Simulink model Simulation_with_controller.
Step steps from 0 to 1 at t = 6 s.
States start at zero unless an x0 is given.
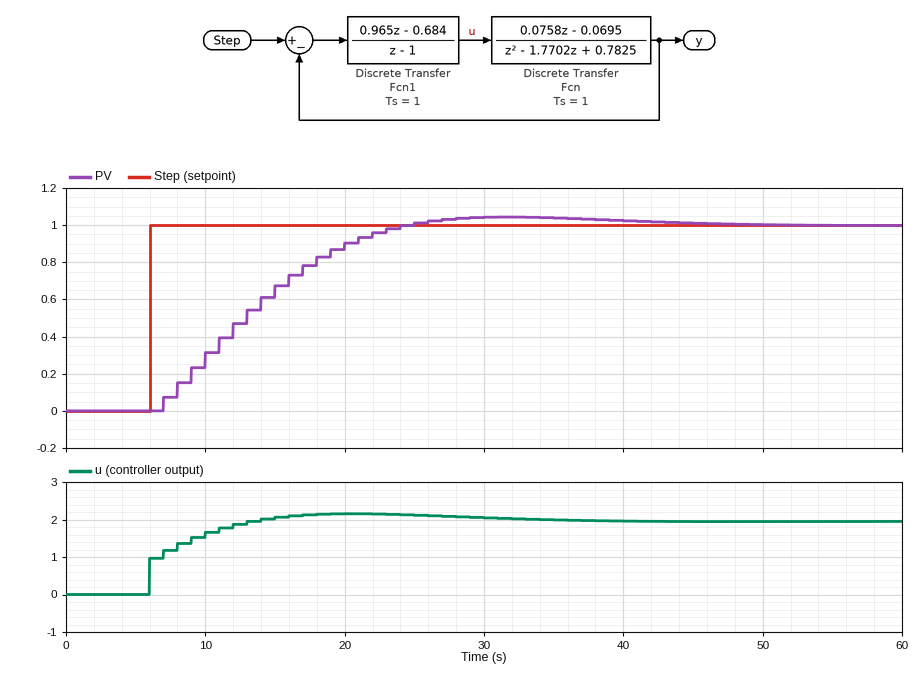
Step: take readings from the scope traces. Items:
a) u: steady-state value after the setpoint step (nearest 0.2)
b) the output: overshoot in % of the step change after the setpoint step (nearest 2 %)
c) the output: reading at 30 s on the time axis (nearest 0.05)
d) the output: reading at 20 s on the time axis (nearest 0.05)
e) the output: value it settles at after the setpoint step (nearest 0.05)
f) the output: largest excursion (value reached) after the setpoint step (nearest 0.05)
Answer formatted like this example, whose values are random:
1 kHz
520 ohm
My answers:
2.0
4 %
1.05
0.90
1.00
1.05
